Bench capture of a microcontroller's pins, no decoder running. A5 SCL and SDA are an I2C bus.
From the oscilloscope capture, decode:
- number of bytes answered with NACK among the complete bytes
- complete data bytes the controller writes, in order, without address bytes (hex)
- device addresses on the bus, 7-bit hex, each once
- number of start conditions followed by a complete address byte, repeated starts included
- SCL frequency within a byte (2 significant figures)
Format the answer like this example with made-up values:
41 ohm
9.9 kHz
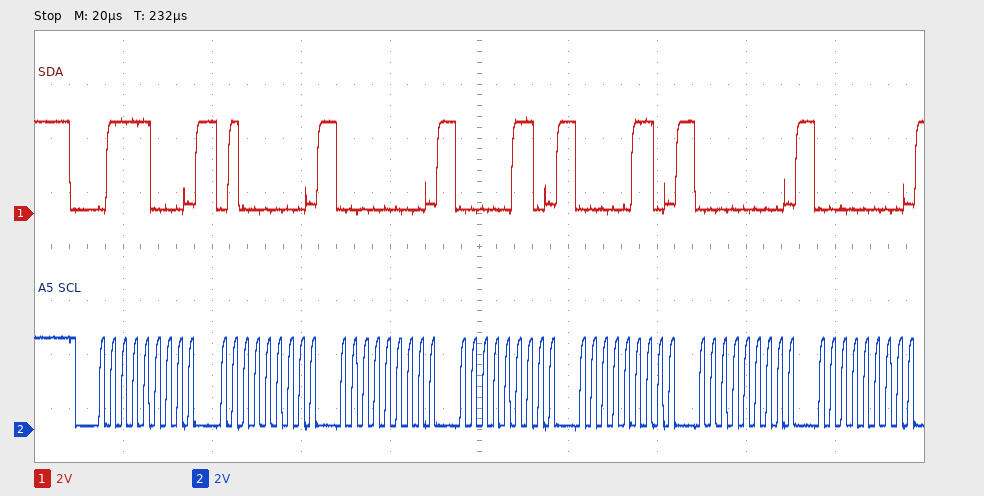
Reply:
0
40 00 06 06 00 00
0x3C
1
400 kHz
